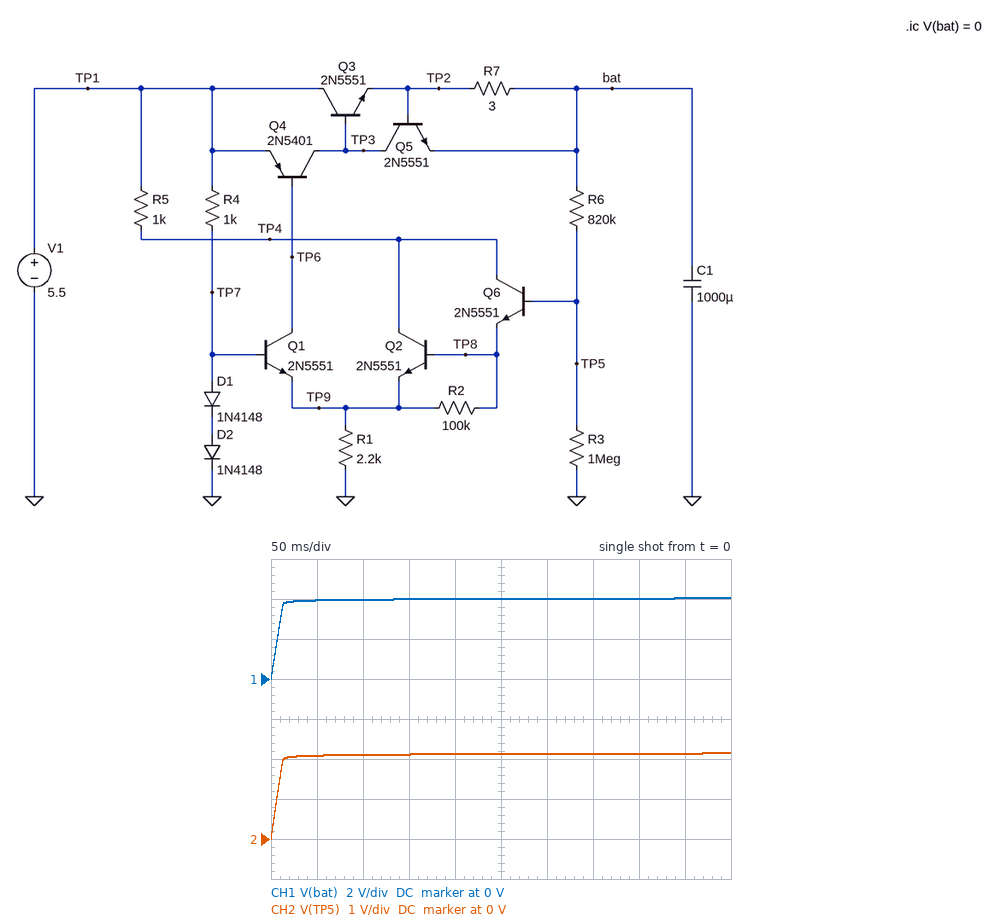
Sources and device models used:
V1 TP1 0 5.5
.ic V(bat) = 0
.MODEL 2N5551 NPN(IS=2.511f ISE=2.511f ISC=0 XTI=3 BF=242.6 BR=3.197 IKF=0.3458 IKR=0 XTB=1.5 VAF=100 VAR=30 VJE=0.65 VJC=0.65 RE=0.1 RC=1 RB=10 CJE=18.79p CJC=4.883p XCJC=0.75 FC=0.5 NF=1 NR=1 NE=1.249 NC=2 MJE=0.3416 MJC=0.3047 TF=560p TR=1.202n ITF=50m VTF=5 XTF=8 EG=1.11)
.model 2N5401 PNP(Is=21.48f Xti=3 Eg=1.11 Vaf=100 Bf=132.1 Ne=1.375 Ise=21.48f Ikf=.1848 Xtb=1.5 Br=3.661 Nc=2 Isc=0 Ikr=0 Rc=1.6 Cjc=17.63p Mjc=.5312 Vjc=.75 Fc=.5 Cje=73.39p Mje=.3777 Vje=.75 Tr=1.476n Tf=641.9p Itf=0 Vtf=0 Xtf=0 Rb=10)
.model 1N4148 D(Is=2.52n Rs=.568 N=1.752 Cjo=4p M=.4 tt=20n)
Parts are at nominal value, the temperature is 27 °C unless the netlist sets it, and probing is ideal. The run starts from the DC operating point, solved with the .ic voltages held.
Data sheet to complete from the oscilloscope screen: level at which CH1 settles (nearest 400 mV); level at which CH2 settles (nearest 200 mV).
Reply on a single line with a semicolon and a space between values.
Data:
4.0 V; 2.2 V
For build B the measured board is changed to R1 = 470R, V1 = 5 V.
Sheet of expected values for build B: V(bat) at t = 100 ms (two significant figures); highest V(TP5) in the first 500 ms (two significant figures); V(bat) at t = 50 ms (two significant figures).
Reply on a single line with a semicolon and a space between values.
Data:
4.2 V; 2.2 V; 4.1 V
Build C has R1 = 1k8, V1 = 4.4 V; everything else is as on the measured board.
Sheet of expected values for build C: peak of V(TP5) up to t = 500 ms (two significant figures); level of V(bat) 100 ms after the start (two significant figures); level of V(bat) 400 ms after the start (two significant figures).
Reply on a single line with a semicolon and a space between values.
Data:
2.0 V; 3.7 V; 3.8 V
